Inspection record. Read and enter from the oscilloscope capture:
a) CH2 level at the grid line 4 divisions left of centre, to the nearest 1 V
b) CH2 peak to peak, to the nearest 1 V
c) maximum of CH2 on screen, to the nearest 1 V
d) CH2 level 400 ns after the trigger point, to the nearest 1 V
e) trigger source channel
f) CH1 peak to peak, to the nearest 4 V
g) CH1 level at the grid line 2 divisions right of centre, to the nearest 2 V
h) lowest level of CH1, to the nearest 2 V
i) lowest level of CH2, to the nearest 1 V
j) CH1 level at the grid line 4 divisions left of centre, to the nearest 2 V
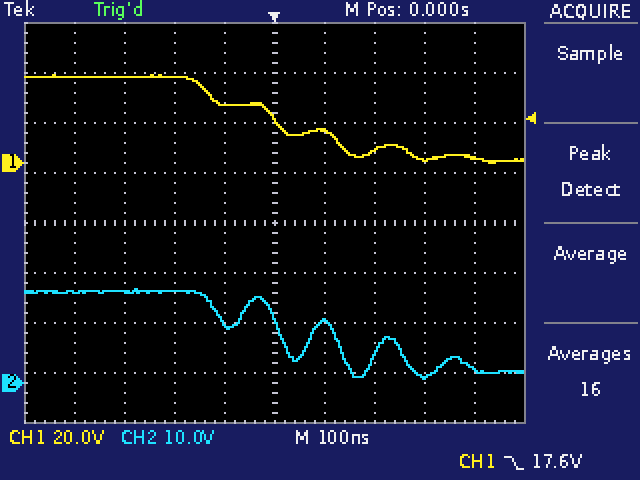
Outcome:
18 V
18 V
19 V
3 V
CH1
36 V
6 V
0 V
1 V
34 V
